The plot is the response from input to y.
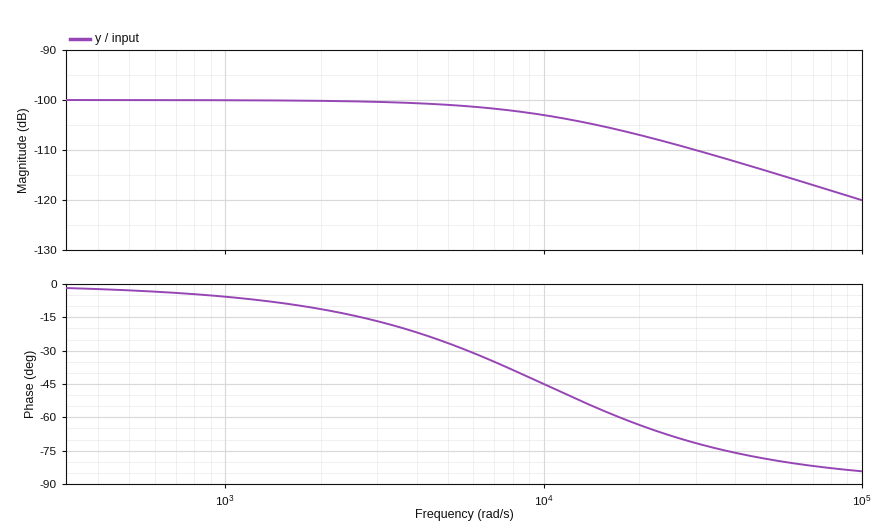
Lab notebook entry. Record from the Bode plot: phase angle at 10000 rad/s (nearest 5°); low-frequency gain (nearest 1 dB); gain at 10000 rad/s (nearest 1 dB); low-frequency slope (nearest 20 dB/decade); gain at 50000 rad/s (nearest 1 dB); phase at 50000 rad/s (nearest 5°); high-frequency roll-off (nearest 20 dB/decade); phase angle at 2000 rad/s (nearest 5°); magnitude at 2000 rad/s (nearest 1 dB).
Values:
-45°
-100 dB
-103 dB
0 dB/decade
-114 dB
-80°
-20 dB/decade
-10°
-100 dB
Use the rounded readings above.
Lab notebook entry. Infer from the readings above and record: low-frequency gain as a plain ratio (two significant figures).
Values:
0.000010
